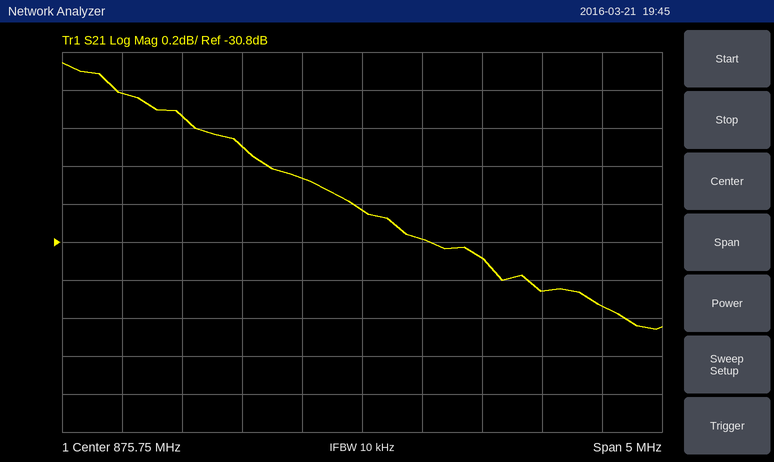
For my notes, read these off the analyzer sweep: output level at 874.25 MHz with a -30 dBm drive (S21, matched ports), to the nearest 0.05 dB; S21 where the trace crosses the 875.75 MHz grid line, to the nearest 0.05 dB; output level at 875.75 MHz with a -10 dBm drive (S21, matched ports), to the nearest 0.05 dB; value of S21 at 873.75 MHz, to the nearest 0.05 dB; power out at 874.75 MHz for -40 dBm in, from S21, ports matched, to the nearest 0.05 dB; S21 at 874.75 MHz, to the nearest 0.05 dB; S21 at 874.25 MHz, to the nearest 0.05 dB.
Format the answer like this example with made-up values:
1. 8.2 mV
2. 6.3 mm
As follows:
1. -60.15 dBm
2. -30.65 dB
3. -40.65 dBm
4. -30.00 dB
5. -70.30 dBm
6. -30.30 dB
7. -30.15 dB
